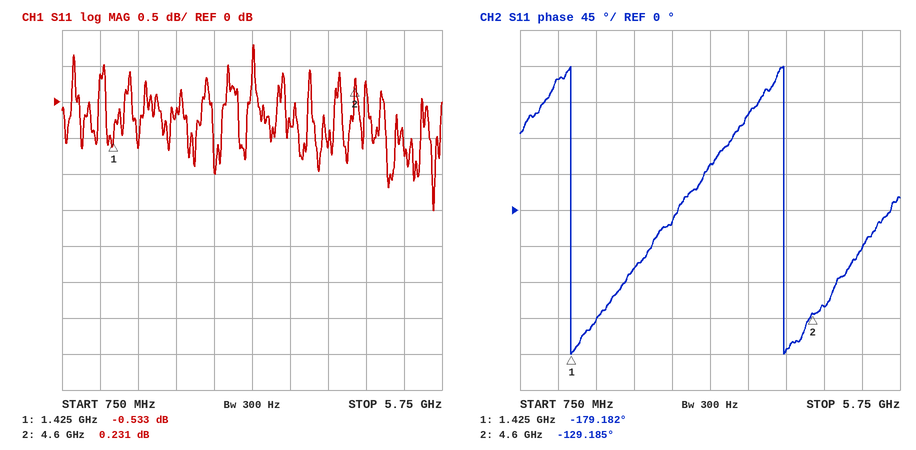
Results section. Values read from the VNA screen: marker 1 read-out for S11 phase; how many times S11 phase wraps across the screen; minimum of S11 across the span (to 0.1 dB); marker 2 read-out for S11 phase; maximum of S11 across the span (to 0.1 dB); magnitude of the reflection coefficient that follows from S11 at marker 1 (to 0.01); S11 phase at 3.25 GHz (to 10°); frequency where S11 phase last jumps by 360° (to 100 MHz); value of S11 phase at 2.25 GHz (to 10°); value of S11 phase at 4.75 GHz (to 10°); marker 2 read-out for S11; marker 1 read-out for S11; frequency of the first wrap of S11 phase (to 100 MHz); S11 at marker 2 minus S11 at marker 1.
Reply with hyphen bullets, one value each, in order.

- -179.182°
- 2
- -1.5 dB
- -129.185°
- 0.8 dB
- 0.94
- 60°
- 4.2 GHz
- -70°
- -120°
- 0.231 dB
- -0.533 dB
- 1.4 GHz
- 0.764 dB
